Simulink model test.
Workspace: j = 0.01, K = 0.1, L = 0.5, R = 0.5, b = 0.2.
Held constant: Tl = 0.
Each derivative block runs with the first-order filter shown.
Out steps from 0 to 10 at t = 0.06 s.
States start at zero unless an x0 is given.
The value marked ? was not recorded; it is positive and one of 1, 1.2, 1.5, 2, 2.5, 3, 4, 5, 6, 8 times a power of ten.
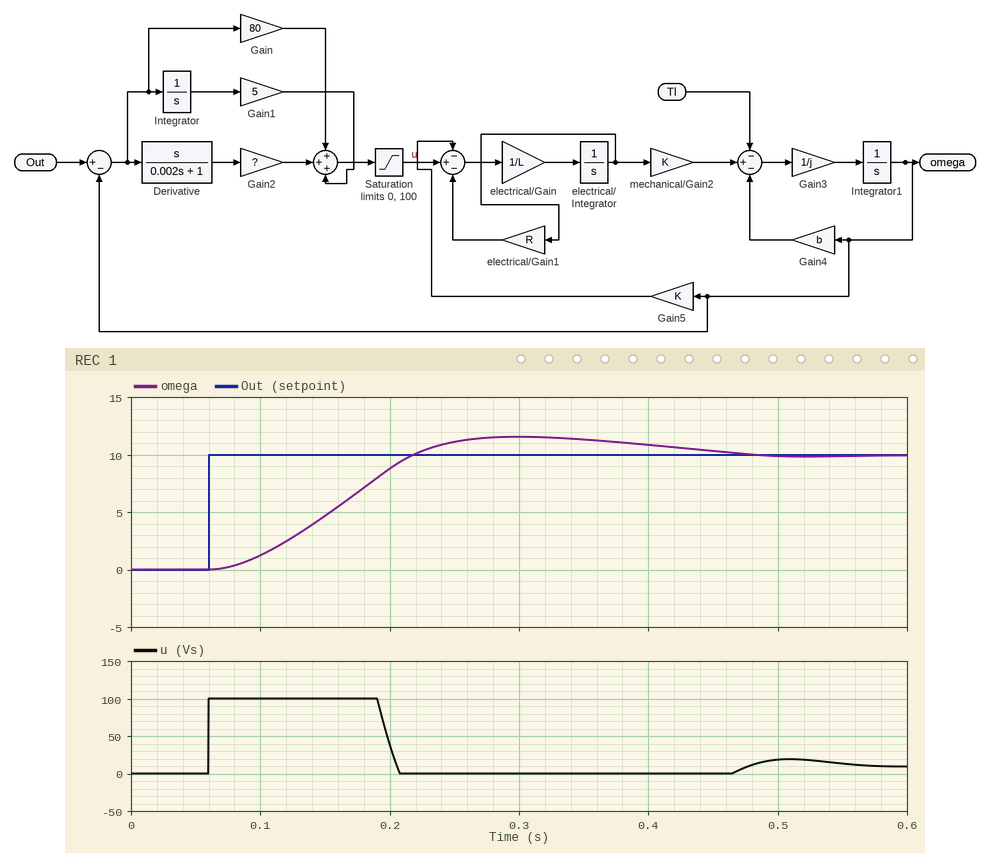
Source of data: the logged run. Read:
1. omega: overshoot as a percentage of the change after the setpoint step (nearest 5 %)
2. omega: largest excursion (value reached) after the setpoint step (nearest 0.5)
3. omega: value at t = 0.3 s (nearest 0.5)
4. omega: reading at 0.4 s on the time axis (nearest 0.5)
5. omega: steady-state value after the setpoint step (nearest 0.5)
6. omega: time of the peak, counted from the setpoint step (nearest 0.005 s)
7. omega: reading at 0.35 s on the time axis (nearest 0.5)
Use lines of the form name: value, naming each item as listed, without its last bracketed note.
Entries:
omega: overshoot as a percentage of the change after the setpoint step: 15 %
omega: largest excursion (value reached) after the setpoint step: 11.5
omega: value at t = 0.3 s: 11.5
omega: reading at 0.4 s on the time axis: 11.0
omega: steady-state value after the setpoint step: 10.0
omega: time of the peak, counted from the setpoint step: 0.240 s
omega: reading at 0.35 s on the time axis: 11.5
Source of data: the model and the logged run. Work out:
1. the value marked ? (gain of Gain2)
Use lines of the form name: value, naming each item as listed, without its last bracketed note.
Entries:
the value marked ?: 0.8
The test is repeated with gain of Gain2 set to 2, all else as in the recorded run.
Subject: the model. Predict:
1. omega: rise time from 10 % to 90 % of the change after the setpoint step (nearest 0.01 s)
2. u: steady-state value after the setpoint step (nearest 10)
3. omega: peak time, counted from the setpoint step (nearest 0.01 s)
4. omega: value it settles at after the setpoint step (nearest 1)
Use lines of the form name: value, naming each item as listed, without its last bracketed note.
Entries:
omega: rise time from 10 % to 90 % of the change after the setpoint step: 0.11 s
u: steady-state value after the setpoint step: 10
omega: peak time, counted from the setpoint step: 0.23 s
omega: value it settles at after the setpoint step: 10
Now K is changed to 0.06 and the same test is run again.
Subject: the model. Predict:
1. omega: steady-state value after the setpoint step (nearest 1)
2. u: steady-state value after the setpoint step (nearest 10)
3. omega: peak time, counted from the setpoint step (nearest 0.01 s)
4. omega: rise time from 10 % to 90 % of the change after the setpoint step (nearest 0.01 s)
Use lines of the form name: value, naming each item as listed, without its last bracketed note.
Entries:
omega: steady-state value after the setpoint step: 10
u: steady-state value after the setpoint step: 20
omega: peak time, counted from the setpoint step: 0.30 s
omega: rise time from 10 % to 90 % of the change after the setpoint step: 0.16 s
